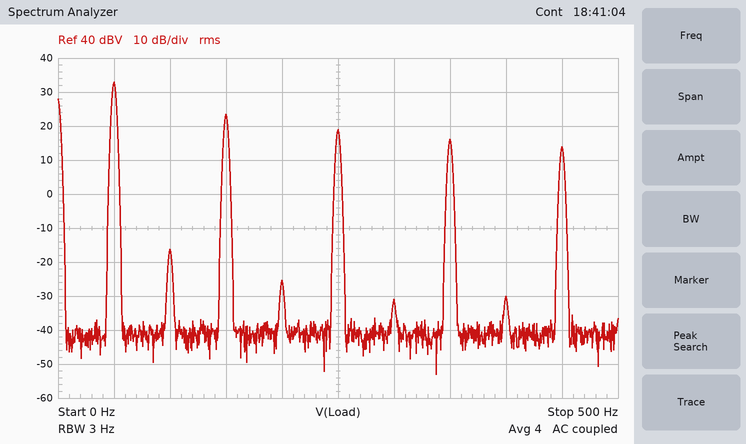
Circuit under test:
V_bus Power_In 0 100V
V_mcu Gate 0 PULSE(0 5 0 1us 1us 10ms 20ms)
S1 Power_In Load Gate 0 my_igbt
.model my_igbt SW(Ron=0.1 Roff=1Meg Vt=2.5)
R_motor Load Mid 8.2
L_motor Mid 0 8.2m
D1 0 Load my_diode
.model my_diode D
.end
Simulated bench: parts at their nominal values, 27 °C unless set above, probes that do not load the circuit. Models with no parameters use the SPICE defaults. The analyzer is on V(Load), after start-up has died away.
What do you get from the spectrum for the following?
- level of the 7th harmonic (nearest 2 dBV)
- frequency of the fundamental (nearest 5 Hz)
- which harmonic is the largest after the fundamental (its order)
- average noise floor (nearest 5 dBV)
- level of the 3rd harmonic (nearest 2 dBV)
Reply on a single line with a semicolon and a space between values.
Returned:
16 dBV; 50 Hz; 3; -40 dBV; 24 dBV
